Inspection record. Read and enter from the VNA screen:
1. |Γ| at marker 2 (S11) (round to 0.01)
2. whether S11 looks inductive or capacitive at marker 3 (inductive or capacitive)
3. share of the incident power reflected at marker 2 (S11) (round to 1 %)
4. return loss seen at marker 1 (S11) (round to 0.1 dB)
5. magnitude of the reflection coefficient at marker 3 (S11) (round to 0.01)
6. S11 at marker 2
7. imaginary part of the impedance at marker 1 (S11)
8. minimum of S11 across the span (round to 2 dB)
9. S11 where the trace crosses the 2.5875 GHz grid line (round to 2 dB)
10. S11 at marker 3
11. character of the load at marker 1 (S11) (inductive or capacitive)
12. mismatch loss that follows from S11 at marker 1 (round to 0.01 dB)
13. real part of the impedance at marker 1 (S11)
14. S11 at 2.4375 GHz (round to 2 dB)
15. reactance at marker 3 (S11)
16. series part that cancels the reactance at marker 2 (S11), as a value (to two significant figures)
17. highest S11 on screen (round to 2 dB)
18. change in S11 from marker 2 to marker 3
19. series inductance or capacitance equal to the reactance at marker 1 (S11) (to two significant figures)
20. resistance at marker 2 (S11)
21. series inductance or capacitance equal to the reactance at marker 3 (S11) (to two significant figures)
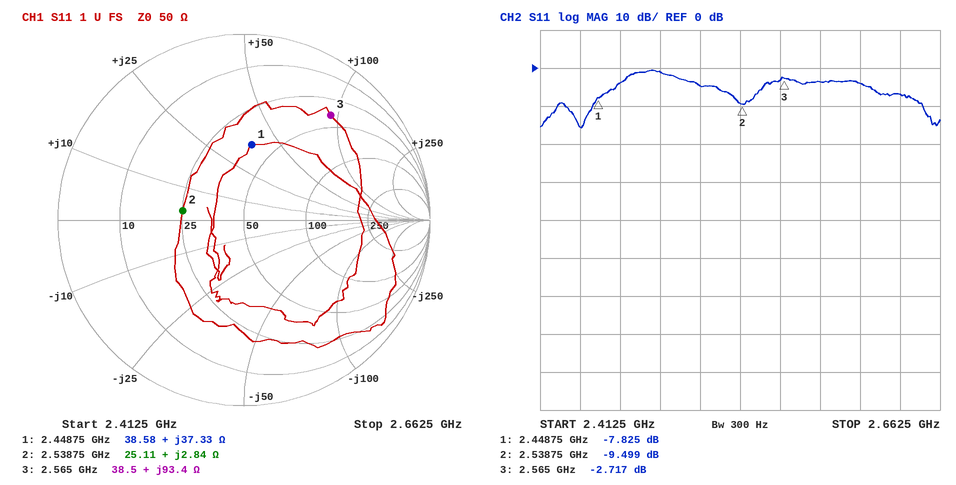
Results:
0.33
inductive
11 %
7.8 dB
0.73
-9.499 dB
+37.33 Ω
-16 dB
-4 dB
-2.717 dB
inductive
0.78 dB
38.58 Ω
-16 dB
+93.4 Ω
22 pF
0 dB
6.782 dB
2.4 nH
25.11 Ω
5.8 nH
